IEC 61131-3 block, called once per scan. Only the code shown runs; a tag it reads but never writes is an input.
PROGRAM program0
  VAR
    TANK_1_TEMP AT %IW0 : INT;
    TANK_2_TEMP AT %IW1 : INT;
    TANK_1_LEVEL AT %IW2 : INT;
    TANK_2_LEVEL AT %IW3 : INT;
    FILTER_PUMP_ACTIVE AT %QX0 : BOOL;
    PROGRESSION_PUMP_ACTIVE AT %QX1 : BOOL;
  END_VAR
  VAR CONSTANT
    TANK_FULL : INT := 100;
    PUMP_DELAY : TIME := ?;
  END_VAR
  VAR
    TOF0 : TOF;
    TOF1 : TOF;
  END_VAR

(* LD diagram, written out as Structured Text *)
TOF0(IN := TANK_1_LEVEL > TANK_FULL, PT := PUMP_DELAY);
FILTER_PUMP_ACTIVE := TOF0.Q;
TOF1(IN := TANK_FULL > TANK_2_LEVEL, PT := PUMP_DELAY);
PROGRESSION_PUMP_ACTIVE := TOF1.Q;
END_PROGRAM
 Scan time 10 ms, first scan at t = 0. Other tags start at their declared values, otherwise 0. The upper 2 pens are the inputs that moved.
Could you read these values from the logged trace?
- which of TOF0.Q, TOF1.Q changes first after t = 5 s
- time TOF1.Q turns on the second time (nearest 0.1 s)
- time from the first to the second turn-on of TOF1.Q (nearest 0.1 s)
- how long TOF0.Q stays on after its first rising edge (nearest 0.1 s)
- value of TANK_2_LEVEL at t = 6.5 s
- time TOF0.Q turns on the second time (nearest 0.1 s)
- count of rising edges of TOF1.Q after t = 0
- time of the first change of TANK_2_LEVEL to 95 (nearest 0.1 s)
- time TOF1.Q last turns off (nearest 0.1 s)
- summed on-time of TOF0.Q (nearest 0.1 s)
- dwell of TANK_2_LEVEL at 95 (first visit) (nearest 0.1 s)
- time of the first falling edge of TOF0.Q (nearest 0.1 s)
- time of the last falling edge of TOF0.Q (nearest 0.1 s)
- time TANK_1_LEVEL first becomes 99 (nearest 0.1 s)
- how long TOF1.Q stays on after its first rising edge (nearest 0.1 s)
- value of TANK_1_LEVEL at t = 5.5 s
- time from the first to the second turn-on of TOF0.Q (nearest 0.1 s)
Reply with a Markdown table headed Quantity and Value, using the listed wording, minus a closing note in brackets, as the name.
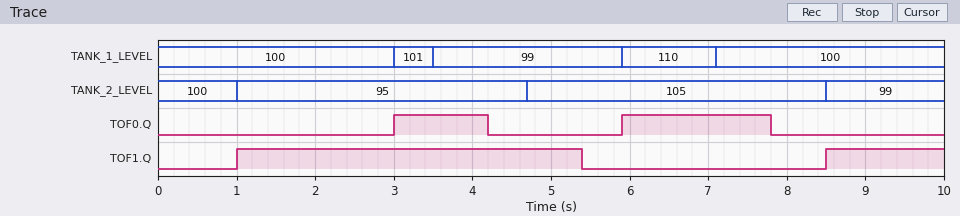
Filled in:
| Quantity | Value |
|---|---|
| which of TOF0.Q, TOF1.Q changes first after t = 5 s | TOF1.Q |
| time TOF1.Q turns on the second time | 8.5 s |
| time from the first to the second turn-on of TOF1.Q | 7.5 s |
| how long TOF0.Q stays on after its first rising edge | 1.2 s |
| value of TANK_2_LEVEL at t = 6.5 s | 105 |
| time TOF0.Q turns on the second time | 5.9 s |
| count of rising edges of TOF1.Q after t = 0 | 2 |
| time of the first change of TANK_2_LEVEL to 95 | 1.0 s |
| time TOF1.Q last turns off | 5.4 s |
| summed on-time of TOF0.Q | 3.1 s |
| dwell of TANK_2_LEVEL at 95 (first visit) | 3.7 s |
| time of the first falling edge of TOF0.Q | 4.2 s |
| time of the last falling edge of TOF0.Q | 7.8 s |
| time TANK_1_LEVEL first becomes 99 | 3.5 s |
| how long TOF1.Q stays on after its first rising edge | 4.4 s |
| value of TANK_1_LEVEL at t = 5.5 s | 99 |
| time from the first to the second turn-on of TOF0.Q | 2.9 s |
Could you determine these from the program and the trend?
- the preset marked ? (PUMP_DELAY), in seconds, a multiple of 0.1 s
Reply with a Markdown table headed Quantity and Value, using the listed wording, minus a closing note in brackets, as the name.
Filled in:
| Quantity | Value |
|---|---|
| the preset marked ? (PUMP_DELAY), in seconds, a multiple of 0.1 s | 0.7 s |
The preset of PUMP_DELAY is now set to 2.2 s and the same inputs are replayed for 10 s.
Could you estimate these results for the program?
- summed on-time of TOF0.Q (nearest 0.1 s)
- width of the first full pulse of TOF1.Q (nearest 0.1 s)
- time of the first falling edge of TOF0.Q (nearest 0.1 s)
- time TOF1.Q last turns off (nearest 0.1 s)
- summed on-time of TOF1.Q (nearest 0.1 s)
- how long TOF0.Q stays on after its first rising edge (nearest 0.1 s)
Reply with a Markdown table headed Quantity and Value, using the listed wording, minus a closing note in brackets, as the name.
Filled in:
| Quantity | Value |
|---|---|
| summed on-time of TOF0.Q | 6.1 s |
| width of the first full pulse of TOF1.Q | 5.9 s |
| time of the first falling edge of TOF0.Q | 5.7 s |
| time TOF1.Q last turns off | 6.9 s |
| summed on-time of TOF1.Q | 7.4 s |
| how long TOF0.Q stays on after its first rising edge | 2.7 s |
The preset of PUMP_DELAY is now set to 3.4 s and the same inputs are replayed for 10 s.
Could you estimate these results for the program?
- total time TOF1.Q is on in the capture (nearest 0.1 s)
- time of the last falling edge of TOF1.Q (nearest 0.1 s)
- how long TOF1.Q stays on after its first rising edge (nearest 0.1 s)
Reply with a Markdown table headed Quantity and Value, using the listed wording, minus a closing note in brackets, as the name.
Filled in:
| Quantity | Value |
|---|---|
| total time TOF1.Q is on in the capture | 8.6 s |
| time of the last falling edge of TOF1.Q | 8.1 s |
| how long TOF1.Q stays on after its first rising edge | 7.1 s |
